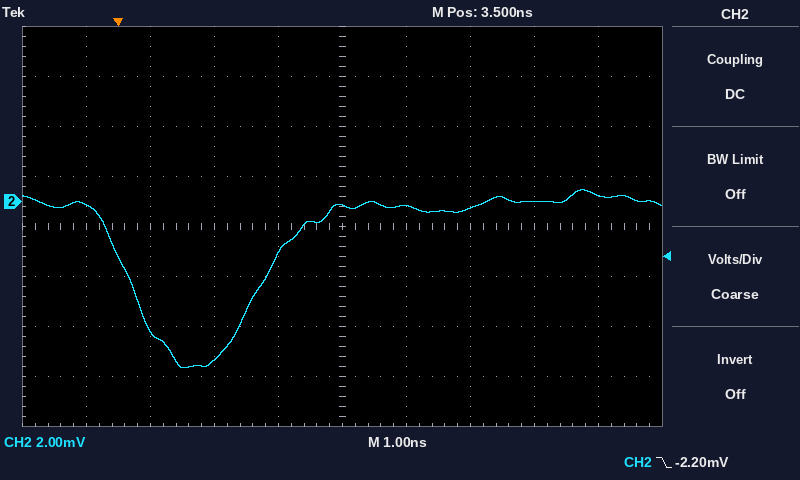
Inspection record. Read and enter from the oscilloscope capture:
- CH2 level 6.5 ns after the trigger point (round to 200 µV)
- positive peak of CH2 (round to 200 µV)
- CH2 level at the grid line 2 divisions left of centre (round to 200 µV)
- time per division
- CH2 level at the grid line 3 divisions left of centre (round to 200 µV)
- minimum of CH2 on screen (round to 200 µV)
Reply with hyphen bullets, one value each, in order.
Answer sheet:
- 0.0 mV
- 400 µV
- -6.4 mV
- 1 ns
- -5.2 mV
- -6.6 mV
